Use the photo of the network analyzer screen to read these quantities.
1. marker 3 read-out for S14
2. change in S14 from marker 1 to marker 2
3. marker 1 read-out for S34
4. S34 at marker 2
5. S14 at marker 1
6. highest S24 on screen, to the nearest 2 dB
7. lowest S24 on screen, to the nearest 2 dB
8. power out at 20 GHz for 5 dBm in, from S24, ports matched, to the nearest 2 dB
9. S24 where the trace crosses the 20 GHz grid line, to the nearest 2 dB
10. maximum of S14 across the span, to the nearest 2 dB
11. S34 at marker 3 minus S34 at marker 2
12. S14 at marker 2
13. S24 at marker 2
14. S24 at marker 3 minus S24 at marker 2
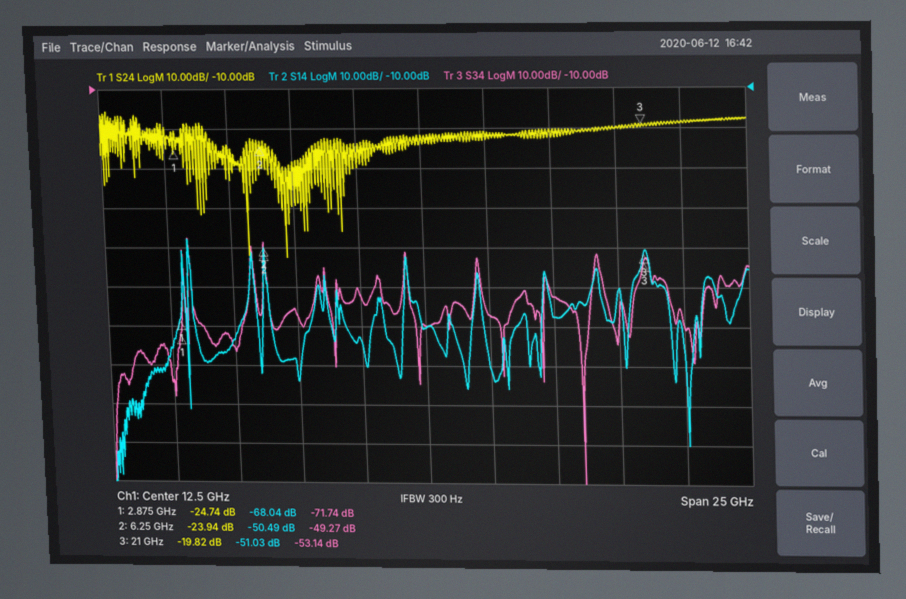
-51.03 dB
17.55 dB
-71.74 dB
-49.27 dB
-68.04 dB
-16 dB
-52 dB
-16 dBm
-20 dB
-48 dB
-3.87 dB
-50.49 dB
-23.94 dB
4.12 dB
